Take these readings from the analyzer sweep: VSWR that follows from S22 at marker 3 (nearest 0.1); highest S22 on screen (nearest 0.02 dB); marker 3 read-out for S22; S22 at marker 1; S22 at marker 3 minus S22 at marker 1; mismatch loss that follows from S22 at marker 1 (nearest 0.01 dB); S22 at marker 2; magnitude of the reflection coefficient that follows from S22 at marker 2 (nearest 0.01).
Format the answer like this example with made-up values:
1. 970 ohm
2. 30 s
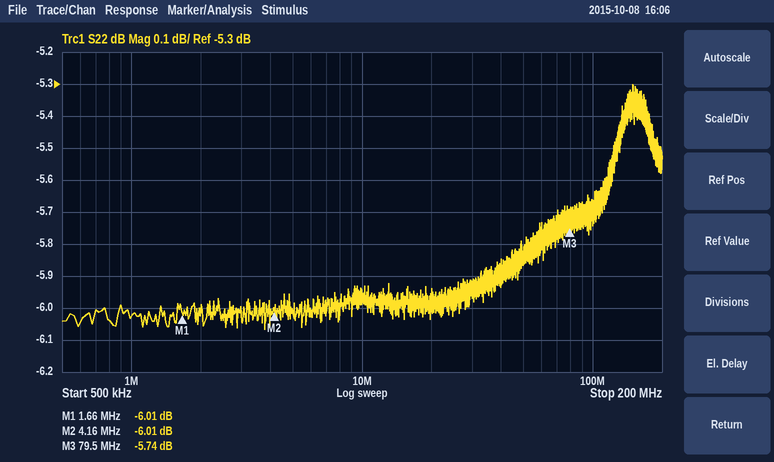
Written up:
1. 3.1
2. -5.30 dB
3. -5.74 dB
4. -6.01 dB
5. 0.27 dB
6. 1.25 dB
7. -6.01 dB
8. 0.50
